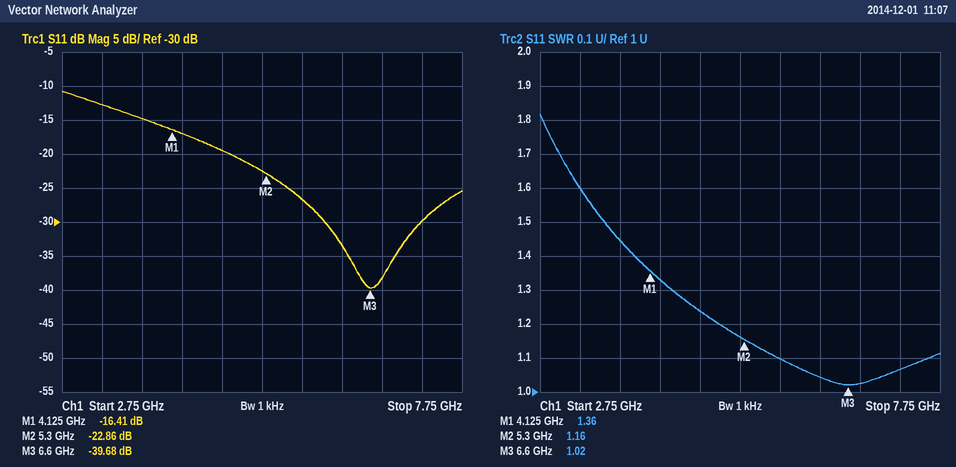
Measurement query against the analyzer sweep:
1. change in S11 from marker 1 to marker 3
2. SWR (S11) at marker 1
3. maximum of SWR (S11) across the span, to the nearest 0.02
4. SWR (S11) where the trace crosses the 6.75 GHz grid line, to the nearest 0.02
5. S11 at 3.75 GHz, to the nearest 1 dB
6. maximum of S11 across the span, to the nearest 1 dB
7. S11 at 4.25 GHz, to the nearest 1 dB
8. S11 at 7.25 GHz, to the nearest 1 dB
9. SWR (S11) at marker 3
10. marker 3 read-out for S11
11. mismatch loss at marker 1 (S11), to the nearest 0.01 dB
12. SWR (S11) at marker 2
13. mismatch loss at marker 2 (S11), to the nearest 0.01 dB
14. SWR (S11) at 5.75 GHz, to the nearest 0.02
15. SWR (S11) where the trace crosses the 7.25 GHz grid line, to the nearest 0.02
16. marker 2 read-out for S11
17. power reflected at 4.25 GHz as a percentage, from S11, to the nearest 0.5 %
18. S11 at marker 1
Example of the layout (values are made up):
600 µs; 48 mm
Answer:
-23.27 dB; 1.36; 1.82; 1.02; -15 dB; -11 dB; -17 dB; -30 dB; 1.02; -39.68 dB; 0.10 dB; 1.16; 0.02 dB; 1.10; 1.06; -22.86 dB; 2.0 %; -16.41 dB
